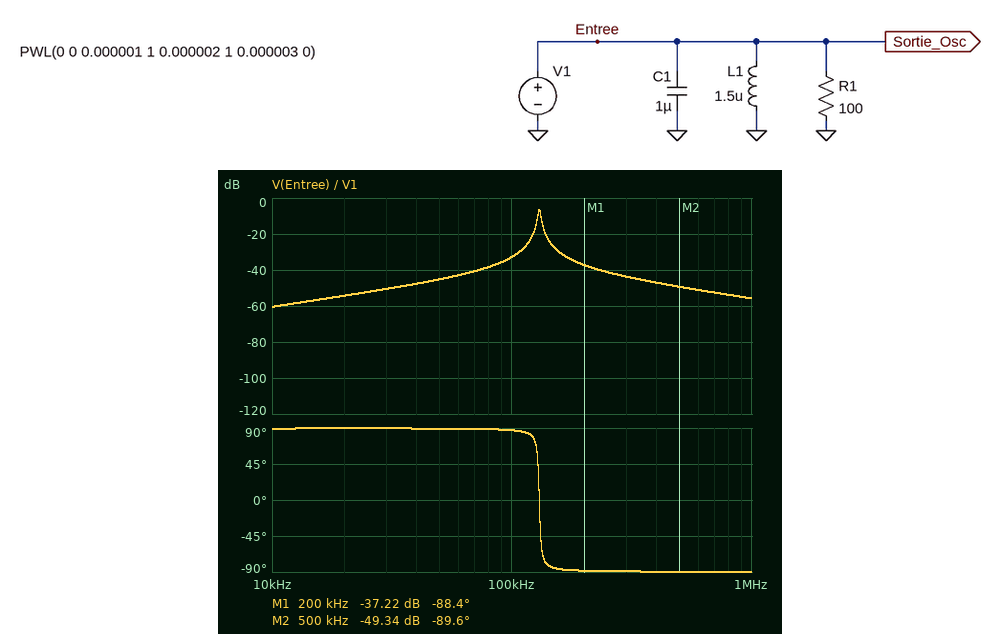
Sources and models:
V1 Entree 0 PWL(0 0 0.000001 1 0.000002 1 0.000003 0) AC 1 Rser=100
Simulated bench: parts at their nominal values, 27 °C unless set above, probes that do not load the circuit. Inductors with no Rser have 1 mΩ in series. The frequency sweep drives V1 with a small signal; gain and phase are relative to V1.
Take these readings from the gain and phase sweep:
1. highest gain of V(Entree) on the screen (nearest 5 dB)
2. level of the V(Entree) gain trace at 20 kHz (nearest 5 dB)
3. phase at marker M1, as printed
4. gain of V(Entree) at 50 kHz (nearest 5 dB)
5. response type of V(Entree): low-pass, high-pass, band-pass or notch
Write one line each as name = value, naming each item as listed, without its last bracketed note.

highest gain of V(Entree) on the screen = -5 dB
level of the V(Entree) gain trace at 20 kHz = -55 dB
phase at marker M1, as printed = -88.4 deg
gain of V(Entree) at 50 kHz = -45 dB
response type of V(Entree): low-pass, high-pass, band-pass or notch = band-pass
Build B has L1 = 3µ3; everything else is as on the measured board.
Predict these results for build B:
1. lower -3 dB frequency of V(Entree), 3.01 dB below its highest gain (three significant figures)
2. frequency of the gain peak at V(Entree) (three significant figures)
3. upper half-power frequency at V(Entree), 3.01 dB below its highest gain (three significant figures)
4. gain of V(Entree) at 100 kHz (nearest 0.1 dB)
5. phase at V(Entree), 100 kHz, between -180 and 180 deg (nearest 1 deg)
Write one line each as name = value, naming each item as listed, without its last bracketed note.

lower -3 dB frequency of V(Entree), 3.01 dB below its highest gain = 86.0 kHz
frequency of the gain peak at V(Entree) = 87.6 kHz
upper half-power frequency at V(Entree), 3.01 dB below its highest gain = 89.2 kHz
gain of V(Entree) at 100 kHz = -23.4 dB
phase at V(Entree), 100 kHz, between -180 and 180 deg = -82 deg
